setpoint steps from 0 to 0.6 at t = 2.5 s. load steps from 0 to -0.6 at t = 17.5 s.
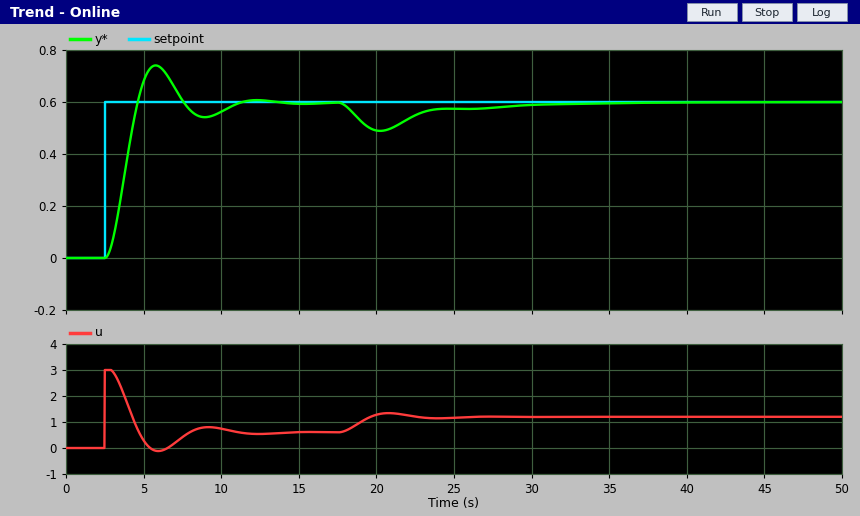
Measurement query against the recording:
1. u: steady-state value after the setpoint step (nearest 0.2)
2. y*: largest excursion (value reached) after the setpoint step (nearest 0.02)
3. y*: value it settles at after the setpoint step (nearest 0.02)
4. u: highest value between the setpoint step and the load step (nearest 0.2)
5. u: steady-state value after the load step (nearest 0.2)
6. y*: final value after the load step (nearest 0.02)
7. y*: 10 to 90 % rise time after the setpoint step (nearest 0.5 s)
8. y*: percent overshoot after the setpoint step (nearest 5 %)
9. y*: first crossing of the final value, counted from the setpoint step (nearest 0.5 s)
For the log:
0.6
0.74
0.60
3.0
1.2
0.60
1.5 s
25 %
2.0 s
